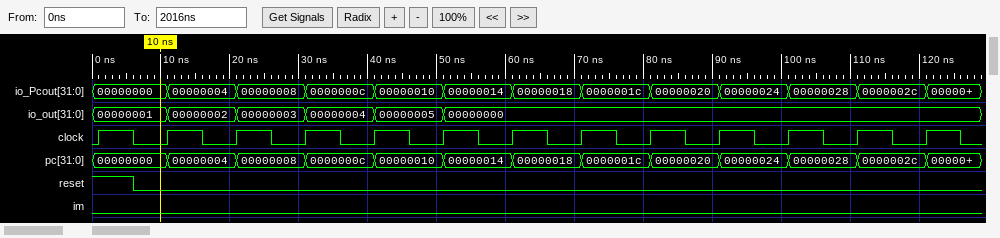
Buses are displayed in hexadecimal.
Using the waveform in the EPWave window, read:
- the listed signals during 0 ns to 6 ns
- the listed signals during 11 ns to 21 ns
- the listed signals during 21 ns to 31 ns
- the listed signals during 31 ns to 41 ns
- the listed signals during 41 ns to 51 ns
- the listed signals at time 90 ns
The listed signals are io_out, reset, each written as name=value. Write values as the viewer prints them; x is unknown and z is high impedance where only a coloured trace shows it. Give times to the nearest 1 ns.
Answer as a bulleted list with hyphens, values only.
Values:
- io_out=00000001, reset=1
- io_out=00000002, reset=0
- io_out=00000003, reset=0
- io_out=00000004, reset=0
- io_out=00000005, reset=0
- io_out=00000000, reset=0
